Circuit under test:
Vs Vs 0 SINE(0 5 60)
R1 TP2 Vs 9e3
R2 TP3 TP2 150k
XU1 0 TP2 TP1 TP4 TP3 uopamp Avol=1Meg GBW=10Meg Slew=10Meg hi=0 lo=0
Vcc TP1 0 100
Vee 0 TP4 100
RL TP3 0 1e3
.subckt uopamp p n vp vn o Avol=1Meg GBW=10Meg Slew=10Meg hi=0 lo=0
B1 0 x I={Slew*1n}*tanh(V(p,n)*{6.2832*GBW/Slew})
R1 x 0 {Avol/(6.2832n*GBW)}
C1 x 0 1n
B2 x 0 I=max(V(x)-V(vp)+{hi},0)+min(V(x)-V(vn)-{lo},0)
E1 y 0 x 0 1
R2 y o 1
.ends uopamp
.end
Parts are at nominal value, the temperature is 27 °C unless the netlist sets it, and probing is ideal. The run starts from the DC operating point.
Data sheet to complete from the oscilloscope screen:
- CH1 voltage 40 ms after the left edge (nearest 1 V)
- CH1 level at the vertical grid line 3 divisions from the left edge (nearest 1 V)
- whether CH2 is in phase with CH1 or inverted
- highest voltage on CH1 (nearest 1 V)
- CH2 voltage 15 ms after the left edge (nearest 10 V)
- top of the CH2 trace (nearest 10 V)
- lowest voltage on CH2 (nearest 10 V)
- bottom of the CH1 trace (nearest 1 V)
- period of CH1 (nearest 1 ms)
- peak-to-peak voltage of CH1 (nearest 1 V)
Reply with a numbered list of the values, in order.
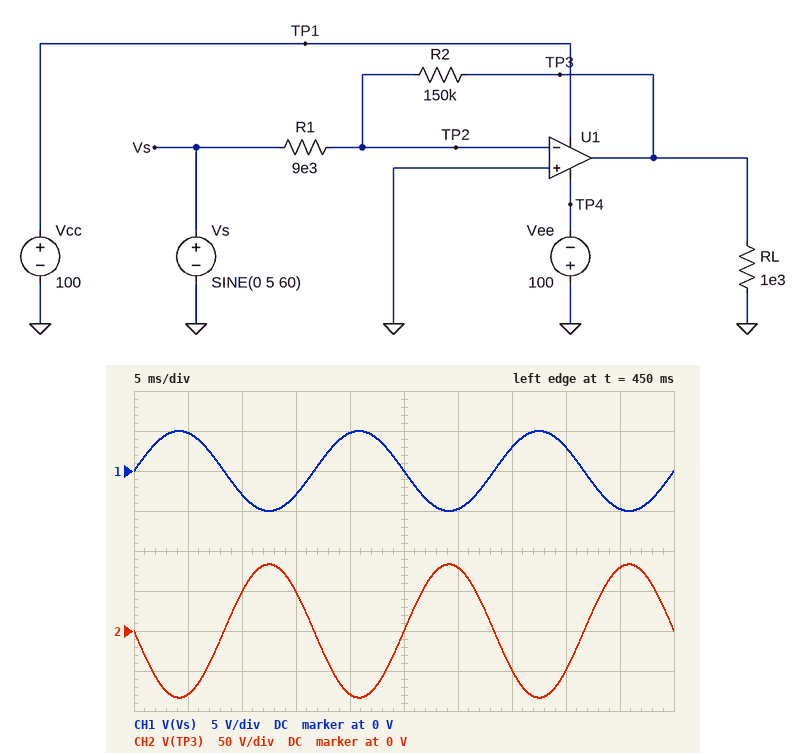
1. 3 V
2. -3 V
3. inverted
4. 5 V
5. 50 V
6. 80 V
7. -80 V
8. -5 V
9. 17 ms
10. 10 V
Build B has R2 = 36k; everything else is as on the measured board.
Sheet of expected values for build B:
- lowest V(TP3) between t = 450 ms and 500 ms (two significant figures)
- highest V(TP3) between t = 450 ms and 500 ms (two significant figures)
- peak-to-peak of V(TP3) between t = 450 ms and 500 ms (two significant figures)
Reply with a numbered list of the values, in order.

1. -20 V
2. 20 V
3. 40 V
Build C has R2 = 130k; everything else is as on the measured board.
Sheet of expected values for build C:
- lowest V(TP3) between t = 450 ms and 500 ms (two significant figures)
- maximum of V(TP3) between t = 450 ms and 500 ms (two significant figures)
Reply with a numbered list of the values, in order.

1. -72 V
2. 72 V
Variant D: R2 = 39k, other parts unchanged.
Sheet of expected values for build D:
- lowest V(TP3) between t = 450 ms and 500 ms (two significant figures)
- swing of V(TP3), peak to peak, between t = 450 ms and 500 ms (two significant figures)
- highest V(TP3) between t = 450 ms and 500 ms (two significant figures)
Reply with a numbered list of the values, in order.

1. -22 V
2. 43 V
3. 22 V
